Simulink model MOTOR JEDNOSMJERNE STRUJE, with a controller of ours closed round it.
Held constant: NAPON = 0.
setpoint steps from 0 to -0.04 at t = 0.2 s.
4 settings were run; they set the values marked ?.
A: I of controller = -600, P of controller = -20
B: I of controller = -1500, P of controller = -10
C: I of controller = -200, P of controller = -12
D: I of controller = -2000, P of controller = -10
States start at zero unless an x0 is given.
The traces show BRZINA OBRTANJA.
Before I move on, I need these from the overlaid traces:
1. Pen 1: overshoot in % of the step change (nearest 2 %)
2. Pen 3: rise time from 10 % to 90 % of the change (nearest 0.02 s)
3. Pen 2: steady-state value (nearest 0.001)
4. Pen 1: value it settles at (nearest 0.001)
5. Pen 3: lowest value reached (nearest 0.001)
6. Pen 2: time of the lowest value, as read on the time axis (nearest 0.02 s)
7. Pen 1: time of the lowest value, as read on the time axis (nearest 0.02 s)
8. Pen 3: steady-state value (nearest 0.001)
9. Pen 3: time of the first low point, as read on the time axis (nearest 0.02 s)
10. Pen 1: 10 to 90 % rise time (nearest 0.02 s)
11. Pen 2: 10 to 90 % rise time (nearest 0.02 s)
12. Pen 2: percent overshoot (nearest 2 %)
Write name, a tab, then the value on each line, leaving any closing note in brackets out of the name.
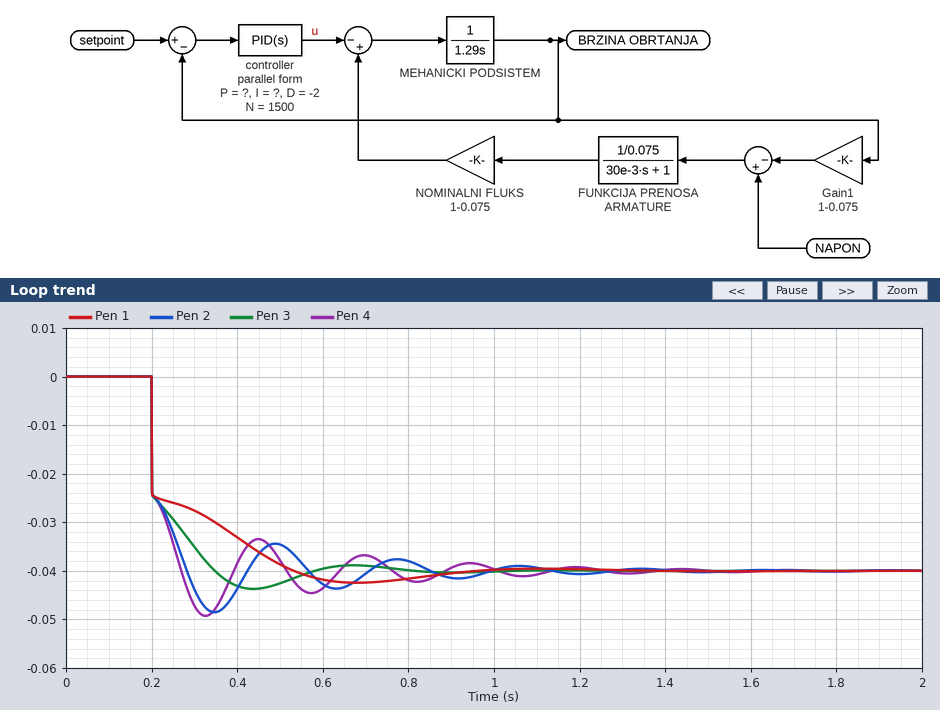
Pen 1: overshoot in % of the step change	6 %
Pen 3: rise time from 10 % to 90 % of the change	0.10 s
Pen 2: steady-state value	-0.040
Pen 1: value it settles at	-0.040
Pen 3: lowest value reached	-0.044
Pen 2: time of the lowest value, as read on the time axis	0.34 s
Pen 1: time of the lowest value, as read on the time axis	0.68 s
Pen 3: steady-state value	-0.040
Pen 3: time of the first low point, as read on the time axis	0.44 s
Pen 1: 10 to 90 % rise time	0.24 s
Pen 2: 10 to 90 % rise time	0.06 s
Pen 2: percent overshoot	22 %
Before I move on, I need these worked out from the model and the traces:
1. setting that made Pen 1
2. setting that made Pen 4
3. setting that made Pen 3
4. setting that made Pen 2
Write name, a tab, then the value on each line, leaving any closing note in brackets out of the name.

setting that made Pen 1	C
setting that made Pen 4	D
setting that made Pen 3	A
setting that made Pen 2	B
